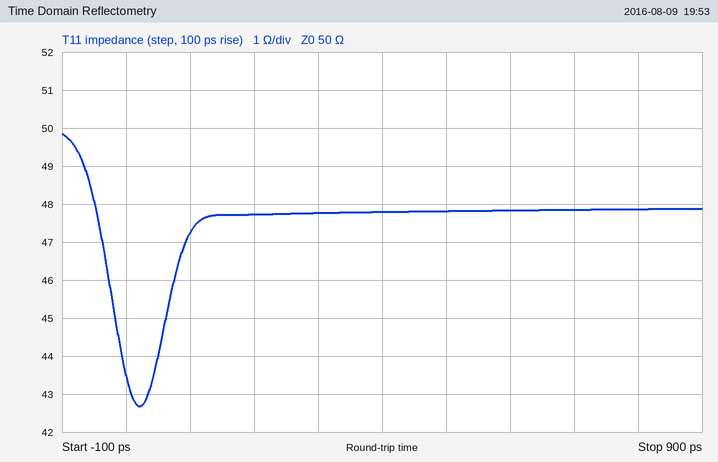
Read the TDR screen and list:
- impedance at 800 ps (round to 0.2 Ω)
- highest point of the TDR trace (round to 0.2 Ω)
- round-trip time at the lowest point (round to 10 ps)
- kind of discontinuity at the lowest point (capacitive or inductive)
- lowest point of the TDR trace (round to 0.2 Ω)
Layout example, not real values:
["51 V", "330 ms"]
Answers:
["47.8 Ω", "49.8 Ω", "20 ps", "capacitive", "42.6 Ω"]
